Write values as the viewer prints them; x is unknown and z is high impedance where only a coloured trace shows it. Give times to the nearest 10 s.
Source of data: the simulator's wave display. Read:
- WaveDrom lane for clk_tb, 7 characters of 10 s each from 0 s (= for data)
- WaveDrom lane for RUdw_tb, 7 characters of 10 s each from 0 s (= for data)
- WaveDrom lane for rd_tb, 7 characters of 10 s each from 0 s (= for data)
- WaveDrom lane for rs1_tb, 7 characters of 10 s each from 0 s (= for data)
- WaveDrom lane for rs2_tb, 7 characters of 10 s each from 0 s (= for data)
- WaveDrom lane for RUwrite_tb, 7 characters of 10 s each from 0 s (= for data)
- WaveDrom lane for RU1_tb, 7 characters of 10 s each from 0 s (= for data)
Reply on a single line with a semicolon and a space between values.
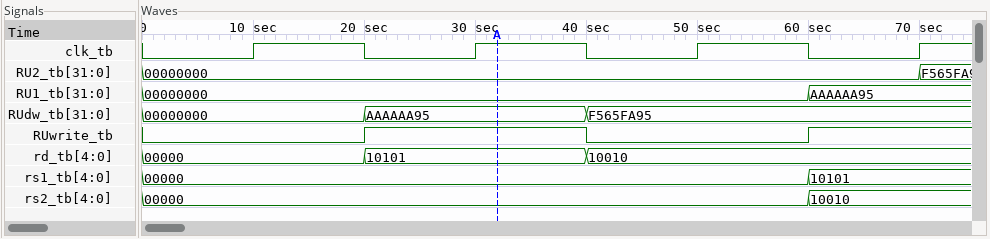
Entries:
{name: 'clk_tb', wave: '0101010'}; {name: 'RUdw_tb', wave: '=.=.=..', data: '00000000 AAAAAA95 F565FA95'}; {name: 'rd_tb', wave: '=.=.=..', data: '00000 10101 10010'}; {name: 'rs1_tb', wave: '=.....=', data: '00000 10101'}; {name: 'rs2_tb', wave: '=.....=', data: '00000 10010'}; {name: 'RUwrite_tb', wave: '0.1.0.1'}; {name: 'RU1_tb', wave: '=.....=', data: '00000000 AAAAAA95'}
